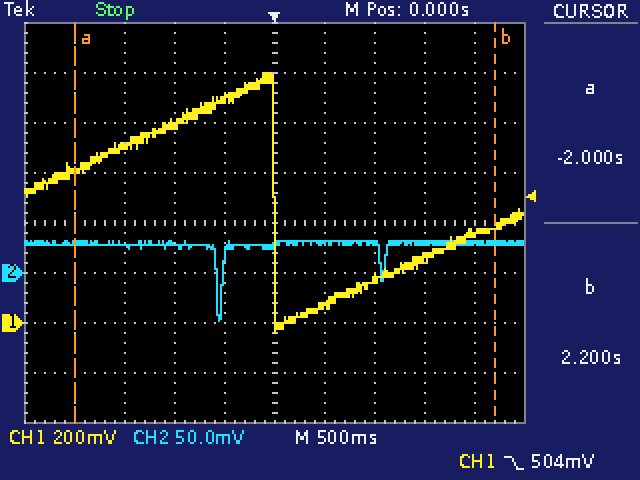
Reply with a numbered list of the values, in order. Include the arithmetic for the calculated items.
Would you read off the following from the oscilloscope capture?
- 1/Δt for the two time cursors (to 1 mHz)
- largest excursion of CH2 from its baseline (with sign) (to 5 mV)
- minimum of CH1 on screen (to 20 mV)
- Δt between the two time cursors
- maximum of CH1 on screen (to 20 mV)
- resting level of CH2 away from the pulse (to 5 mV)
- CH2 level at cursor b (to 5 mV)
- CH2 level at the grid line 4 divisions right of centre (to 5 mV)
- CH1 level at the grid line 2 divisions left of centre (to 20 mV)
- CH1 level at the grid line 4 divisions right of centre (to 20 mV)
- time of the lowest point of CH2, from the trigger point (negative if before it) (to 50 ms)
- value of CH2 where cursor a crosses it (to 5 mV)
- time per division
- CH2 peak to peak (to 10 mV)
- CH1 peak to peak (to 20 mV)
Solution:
1. 1 / 4.20 s ≈ 238 mHz
2. -80 mV
3. -40 mV
4. 2.2 s − (-2 s) = 4.20 s
5. 1.00 V
6. 30 mV
7. 30 mV
8. 30 mV
9. 800 mV
10. 360 mV
11. -550 ms
12. 30 mV
13. 500 ms
14. 80 mV
15. 1.00 V − (-40 mV) = 1.04 V
